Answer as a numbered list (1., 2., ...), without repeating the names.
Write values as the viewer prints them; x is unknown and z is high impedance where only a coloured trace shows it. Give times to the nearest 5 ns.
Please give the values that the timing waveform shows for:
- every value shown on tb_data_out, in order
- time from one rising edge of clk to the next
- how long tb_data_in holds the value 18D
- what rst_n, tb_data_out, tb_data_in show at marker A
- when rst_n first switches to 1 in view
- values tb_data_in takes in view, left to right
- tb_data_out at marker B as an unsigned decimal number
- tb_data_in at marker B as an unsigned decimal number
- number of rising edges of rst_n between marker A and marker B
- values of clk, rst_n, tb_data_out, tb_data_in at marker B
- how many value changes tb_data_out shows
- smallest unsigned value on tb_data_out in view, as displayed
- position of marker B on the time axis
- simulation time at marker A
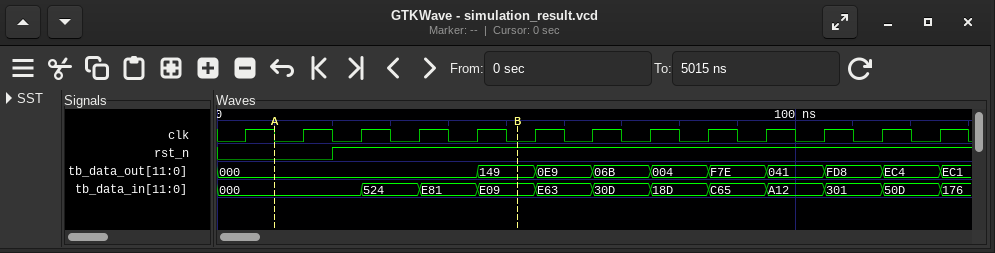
1. 000, 149, 0E9, 06B, 004, F7E, 041, FD8, EC4, EC1
2. 10 ns
3. 10 ns
4. rst_n=0, tb_data_out=000, tb_data_in=000
5. 20 ns
6. 000, 524, E81, E09, E63, 30D, 18D, C65, A12, 301, 50D, 176
7. 329
8. 3593
9. 1
10. clk=0, rst_n=1, tb_data_out=149, tb_data_in=E09
11. 9
12. 000
13. 50 ns
14. 10 ns
